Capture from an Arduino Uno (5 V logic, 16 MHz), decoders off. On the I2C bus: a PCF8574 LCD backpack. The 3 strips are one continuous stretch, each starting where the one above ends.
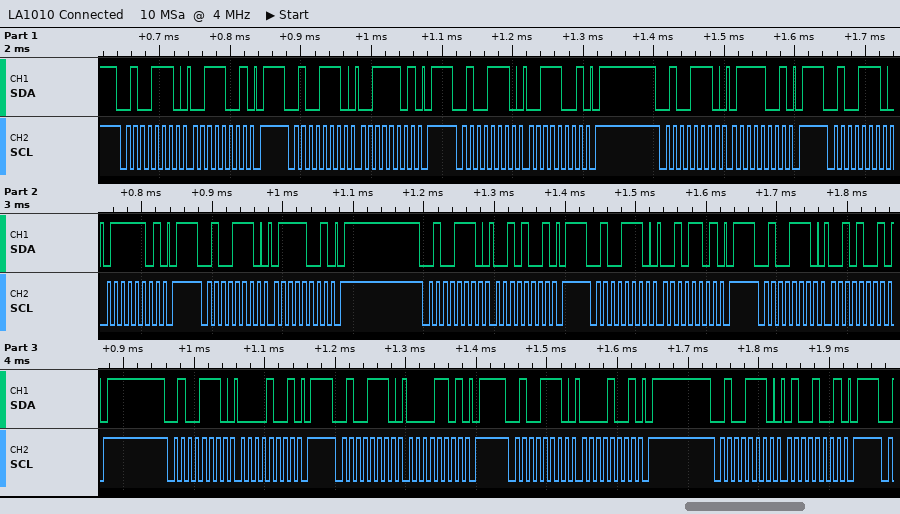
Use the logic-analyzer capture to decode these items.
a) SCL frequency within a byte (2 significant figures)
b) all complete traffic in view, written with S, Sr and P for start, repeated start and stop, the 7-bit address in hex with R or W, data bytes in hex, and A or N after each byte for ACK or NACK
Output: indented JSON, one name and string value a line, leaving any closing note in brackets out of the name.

{
  "SCL frequency within a byte": "100 kHz",
  "all complete traffic in view, written with S, Sr and P for start, repeated start and stop, the 7-bit address in hex with R or W, data bytes in hex, and A or N after each byte for ACK or NACK": "S 27W A 39 A P S 27W A 3D A P S 27W A 39 A P S 27W A 79 A P S 27W A 7D A P S 27W A 79 A P S 27W A 29 A P S 27W A 2D A P S 27W A 29 A P S 27W A 09 A P S 27W A 0D A P S 27W A 09 A P S 27W A 49 A P"
}
